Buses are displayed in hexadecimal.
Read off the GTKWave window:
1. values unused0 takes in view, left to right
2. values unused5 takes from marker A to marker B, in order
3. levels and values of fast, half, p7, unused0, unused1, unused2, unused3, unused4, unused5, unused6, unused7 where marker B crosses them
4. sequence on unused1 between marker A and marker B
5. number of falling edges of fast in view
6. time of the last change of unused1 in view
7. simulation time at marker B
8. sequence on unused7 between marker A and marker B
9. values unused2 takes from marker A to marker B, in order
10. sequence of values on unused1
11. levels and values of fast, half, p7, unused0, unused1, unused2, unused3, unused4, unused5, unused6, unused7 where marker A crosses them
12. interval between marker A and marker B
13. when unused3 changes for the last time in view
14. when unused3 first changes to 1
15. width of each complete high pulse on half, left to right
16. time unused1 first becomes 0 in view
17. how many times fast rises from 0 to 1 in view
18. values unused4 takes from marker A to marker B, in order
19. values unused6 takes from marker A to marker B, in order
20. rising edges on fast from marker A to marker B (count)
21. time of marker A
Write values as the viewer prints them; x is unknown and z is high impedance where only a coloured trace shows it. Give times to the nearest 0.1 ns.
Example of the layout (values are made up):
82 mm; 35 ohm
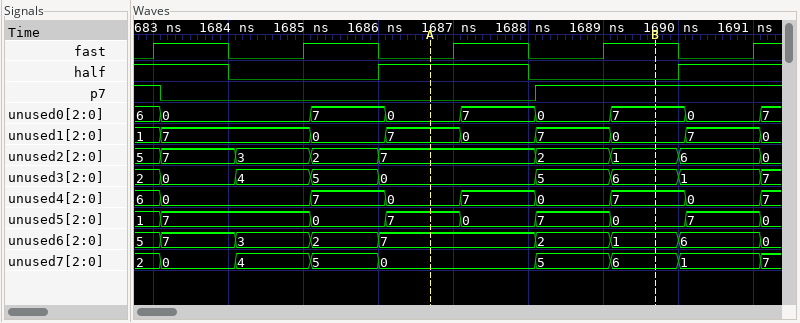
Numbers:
6, 0, 7, 0, 7, 0, 7, 0, 7; 7, 0, 7, 0; fast=1, half=0, p7=1, unused0=7, unused1=0, unused2=1, unused3=6, unused4=7, unused5=0, unused6=1, unused7=6; 7, 0, 7, 0; 4; 1691.1 ns; 1689.7 ns; 0, 5, 6; 7, 2, 1; 1, 7, 0, 7, 0, 7, 0, 7, 0; fast=0, half=1, p7=0, unused0=0, unused1=7, unused2=7, unused3=0, unused4=0, unused5=7, unused6=7, unused7=0; 3 ns; 1691.1 ns; 1690 ns; 2 ns; 1685.1 ns; 5; 0, 7, 0, 7; 7, 2, 1; 2; 1686.7 ns
